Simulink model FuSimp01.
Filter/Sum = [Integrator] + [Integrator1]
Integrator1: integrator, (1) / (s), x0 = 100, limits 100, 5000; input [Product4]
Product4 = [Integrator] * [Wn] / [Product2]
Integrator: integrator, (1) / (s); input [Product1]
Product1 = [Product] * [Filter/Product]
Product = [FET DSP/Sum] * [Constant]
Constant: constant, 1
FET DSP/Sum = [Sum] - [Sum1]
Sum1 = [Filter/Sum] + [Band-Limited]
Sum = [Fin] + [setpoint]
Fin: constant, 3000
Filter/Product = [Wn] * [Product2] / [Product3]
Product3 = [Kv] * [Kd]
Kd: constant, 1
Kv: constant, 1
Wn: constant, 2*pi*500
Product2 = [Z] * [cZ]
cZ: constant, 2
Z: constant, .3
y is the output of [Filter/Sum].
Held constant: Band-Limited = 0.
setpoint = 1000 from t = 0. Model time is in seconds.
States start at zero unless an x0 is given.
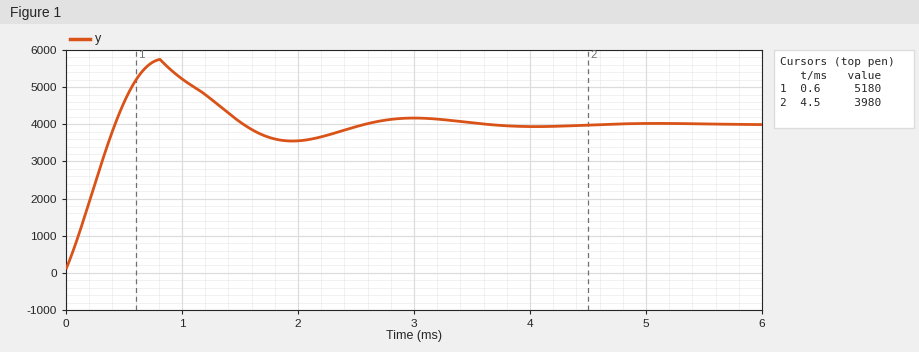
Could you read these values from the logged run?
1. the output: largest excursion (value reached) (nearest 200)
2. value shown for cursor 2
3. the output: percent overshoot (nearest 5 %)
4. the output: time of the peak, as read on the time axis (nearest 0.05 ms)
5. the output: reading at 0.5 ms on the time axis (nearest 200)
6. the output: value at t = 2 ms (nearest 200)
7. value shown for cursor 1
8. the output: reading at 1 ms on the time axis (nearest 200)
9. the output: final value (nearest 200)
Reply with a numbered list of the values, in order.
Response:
1. 5800
2. 3980
3. 45 %
4. 0.80 ms
5. 4600
6. 3600
7. 5180
8. 5200
9. 4000
